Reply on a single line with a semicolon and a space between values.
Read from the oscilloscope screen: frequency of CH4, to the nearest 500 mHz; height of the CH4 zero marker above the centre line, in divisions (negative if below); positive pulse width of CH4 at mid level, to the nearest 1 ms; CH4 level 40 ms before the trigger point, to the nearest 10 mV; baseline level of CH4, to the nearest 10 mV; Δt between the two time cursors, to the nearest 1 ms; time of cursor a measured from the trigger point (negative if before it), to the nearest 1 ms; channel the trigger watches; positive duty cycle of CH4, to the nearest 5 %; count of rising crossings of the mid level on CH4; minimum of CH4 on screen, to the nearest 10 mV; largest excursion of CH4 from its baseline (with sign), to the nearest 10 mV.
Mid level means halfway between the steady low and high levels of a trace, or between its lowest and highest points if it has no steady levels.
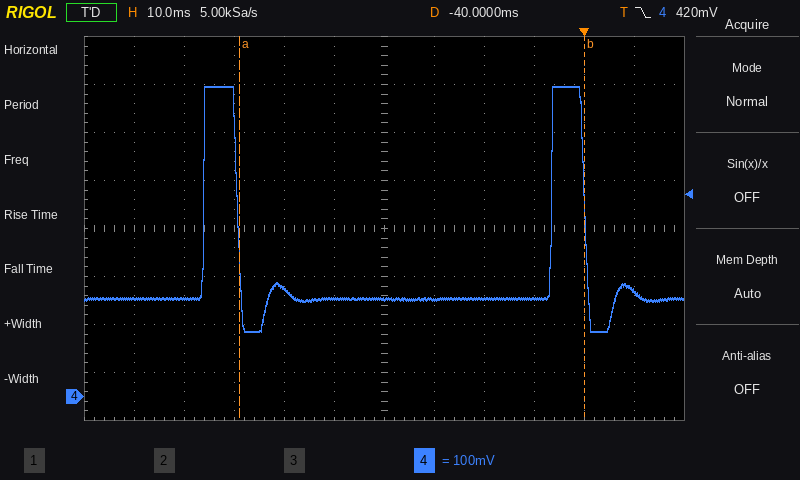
14.5 Hz; -3.5 div; 7 ms; 200 mV; 200 mV; 69 ms; -69 ms; CH4; 10 %; 2; 140 mV; +440 mV
